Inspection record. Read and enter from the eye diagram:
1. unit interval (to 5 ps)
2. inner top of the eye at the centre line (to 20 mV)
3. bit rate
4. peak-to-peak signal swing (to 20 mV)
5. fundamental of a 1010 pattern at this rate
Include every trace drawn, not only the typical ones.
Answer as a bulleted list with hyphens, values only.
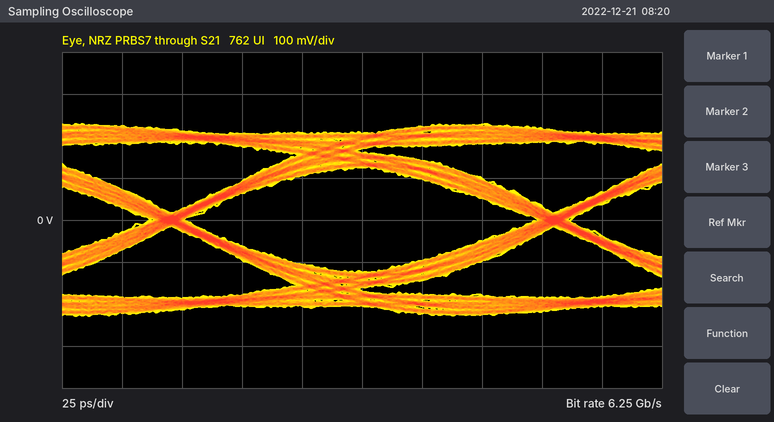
- 160 ps
- 120 mV
- 6.25 Gb/s
- 460 mV
- 3.125 GHz
